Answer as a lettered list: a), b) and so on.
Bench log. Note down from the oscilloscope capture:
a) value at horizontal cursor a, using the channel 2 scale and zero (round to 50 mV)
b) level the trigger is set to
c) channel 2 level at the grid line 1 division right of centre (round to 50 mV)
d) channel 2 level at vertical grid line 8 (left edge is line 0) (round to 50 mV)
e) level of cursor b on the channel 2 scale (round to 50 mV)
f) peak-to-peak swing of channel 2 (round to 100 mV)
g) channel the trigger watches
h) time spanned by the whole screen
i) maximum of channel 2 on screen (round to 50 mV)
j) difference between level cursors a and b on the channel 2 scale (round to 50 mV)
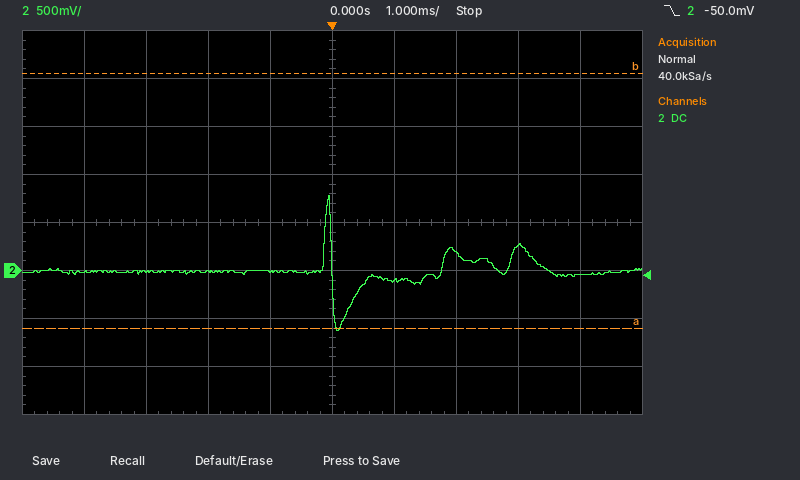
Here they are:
a) -600 mV
b) -50.0 mV
c) -100 mV
d) 250 mV
e) 2.05 V
f) 1.40 V
g) channel 2
h) 10 ms
i) 800 mV
j) 2.65 V
